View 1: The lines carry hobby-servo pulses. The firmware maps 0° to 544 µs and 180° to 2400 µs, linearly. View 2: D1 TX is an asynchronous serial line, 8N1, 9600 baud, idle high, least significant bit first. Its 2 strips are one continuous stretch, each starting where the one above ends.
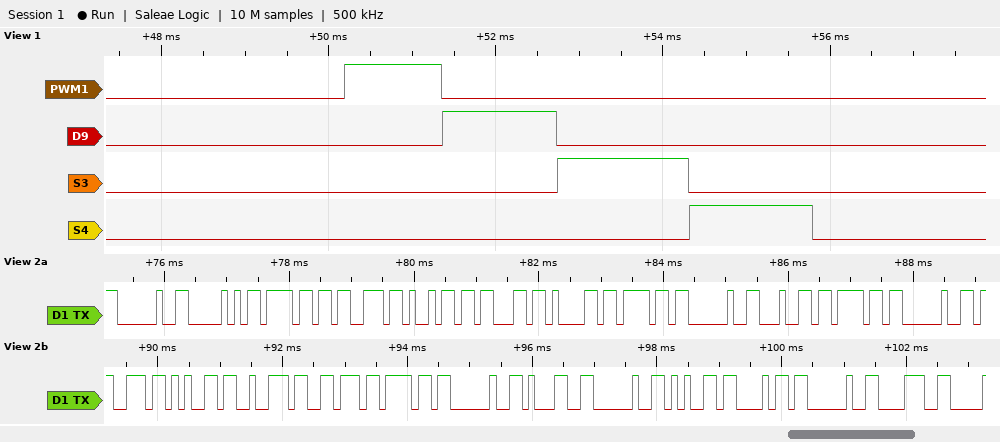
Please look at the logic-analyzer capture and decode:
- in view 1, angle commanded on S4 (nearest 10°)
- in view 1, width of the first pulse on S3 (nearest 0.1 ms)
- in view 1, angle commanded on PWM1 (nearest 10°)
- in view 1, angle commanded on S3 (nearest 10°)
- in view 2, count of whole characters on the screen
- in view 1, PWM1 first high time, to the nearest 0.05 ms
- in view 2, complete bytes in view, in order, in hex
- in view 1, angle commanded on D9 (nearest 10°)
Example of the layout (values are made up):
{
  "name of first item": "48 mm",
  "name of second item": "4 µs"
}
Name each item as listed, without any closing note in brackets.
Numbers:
{
  "in view 1, angle commanded on S4": "90°",
  "in view 1, width of the first pulse on S3": "1.6 ms",
  "in view 1, angle commanded on PWM1": "60°",
  "in view 1, angle commanded on S3": "100°",
  "in view 2, count of whole characters on the screen": "24",
  "in view 1, PWM1 first high time, to the nearest 0.05 ms": "1.15 ms",
  "in view 2, complete bytes in view, in order, in hex": "0x20 0x50 0x6F 0x73 0x69 0x63 0x61 0x6F 0x20 0x64 0x6F 0x20 0x73 0x65 0x72 0x76 0x6F 0x20 0x31 0x20 0x65 0x68 0x20 0x38",
  "in view 1, angle commanded on D9": "80°"
}
